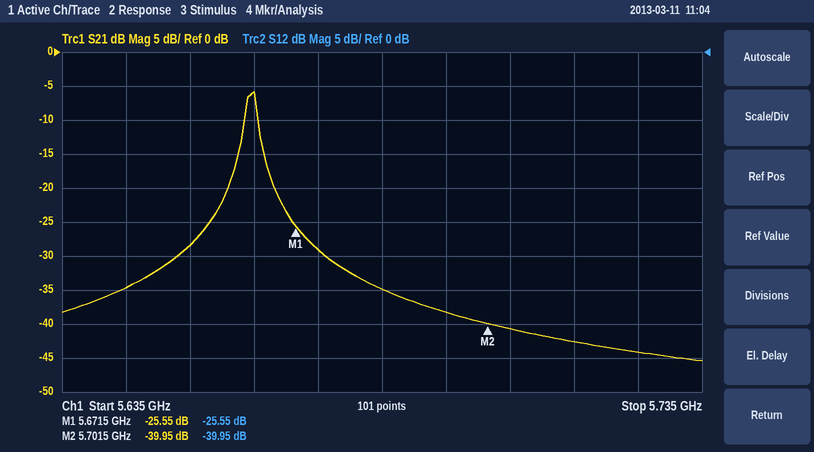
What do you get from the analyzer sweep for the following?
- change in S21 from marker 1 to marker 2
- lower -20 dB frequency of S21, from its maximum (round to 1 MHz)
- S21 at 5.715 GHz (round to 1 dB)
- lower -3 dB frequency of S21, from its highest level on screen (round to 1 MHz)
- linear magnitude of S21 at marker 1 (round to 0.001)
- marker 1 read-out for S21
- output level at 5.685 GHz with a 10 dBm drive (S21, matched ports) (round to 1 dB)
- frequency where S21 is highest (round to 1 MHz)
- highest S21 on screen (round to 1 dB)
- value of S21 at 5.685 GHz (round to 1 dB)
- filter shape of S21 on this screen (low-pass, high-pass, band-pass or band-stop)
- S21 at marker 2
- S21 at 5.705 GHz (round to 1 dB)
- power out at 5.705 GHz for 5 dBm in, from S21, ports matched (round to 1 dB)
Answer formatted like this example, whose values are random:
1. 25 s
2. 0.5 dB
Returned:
1. -14.40 dB
2. 5.657 GHz
3. -43 dB
4. 5.664 GHz
5. 0.053
6. -25.55 dB
7. -25 dBm
8. 5.665 GHz
9. -6 dB
10. -35 dB
11. band-pass
12. -39.95 dB
13. -41 dB
14. -36 dBm
